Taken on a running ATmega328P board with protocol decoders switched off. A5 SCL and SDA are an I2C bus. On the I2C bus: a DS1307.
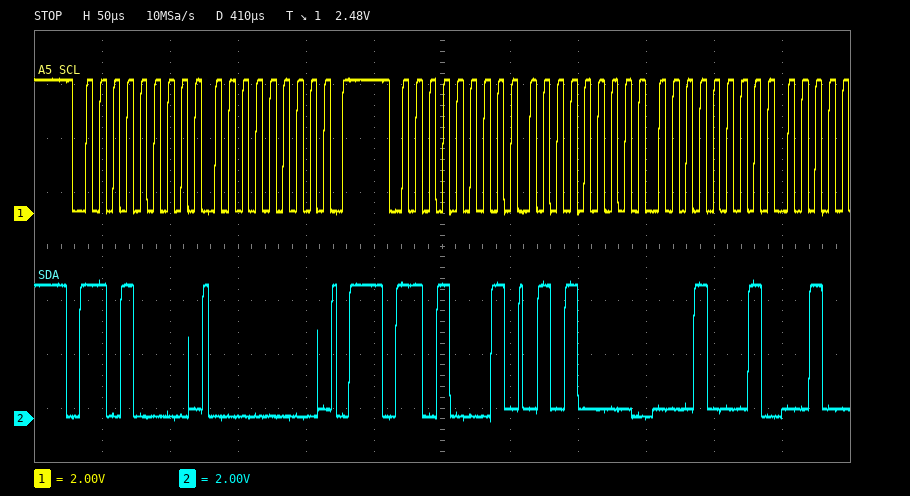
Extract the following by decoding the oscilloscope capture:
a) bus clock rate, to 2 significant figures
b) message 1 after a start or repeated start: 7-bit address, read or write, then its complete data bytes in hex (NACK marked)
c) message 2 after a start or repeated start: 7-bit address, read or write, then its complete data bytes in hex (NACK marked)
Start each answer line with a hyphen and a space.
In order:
- 100 kHz
- 0x68 write: 00
- 0x68 read: 50 11
